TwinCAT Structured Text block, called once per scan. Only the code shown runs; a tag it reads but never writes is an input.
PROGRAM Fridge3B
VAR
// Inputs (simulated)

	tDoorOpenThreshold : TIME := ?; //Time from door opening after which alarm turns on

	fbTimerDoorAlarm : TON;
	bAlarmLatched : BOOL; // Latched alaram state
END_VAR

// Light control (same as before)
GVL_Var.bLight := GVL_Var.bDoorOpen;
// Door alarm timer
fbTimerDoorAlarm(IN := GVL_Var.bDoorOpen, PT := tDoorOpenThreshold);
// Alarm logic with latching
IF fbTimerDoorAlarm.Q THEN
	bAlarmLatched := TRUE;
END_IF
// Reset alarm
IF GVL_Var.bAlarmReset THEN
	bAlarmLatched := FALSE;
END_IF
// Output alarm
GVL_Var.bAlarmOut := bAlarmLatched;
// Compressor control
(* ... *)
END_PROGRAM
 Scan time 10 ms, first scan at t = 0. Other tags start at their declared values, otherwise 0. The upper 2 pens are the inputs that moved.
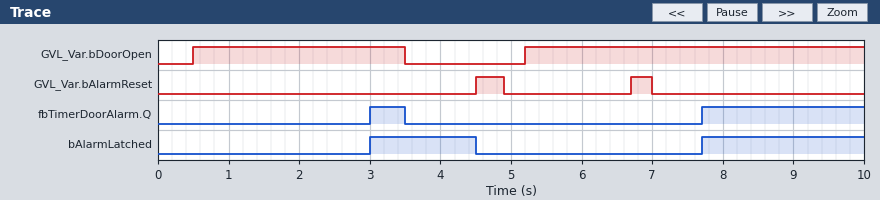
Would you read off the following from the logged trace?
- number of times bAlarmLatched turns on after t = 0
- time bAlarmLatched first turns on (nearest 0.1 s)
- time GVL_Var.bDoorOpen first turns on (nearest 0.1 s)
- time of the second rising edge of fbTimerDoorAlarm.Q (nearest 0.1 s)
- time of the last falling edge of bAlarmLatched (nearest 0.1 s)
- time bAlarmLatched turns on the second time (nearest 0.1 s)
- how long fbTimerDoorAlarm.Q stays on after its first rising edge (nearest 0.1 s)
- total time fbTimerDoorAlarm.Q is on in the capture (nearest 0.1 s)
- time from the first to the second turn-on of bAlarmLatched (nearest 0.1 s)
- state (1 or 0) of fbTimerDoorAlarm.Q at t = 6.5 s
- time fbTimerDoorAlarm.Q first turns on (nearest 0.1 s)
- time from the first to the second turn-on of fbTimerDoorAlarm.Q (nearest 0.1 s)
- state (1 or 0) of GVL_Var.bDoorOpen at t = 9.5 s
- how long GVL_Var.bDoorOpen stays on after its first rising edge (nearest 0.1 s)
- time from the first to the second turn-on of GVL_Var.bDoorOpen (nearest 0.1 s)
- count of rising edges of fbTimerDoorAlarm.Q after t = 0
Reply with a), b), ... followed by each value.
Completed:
a) 2
b) 3.0 s
c) 0.5 s
d) 7.7 s
e) 4.5 s
f) 7.7 s
g) 0.5 s
h) 2.8 s
i) 4.7 s
j) 0
k) 3.0 s
l) 4.7 s
m) 1
n) 3.0 s
o) 4.7 s
p) 2
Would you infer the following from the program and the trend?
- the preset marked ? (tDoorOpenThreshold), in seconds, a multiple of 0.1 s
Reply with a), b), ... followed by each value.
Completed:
a) 2.5 s
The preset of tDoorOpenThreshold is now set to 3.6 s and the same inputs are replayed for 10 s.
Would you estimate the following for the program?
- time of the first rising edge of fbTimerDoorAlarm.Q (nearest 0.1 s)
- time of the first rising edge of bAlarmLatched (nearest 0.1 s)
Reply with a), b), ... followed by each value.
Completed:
a) 8.8 s
b) 8.8 s
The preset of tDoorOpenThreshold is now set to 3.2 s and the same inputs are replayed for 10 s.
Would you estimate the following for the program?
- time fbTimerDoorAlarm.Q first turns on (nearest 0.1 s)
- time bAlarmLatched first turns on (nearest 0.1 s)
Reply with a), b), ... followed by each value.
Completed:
a) 8.4 s
b) 8.4 s
